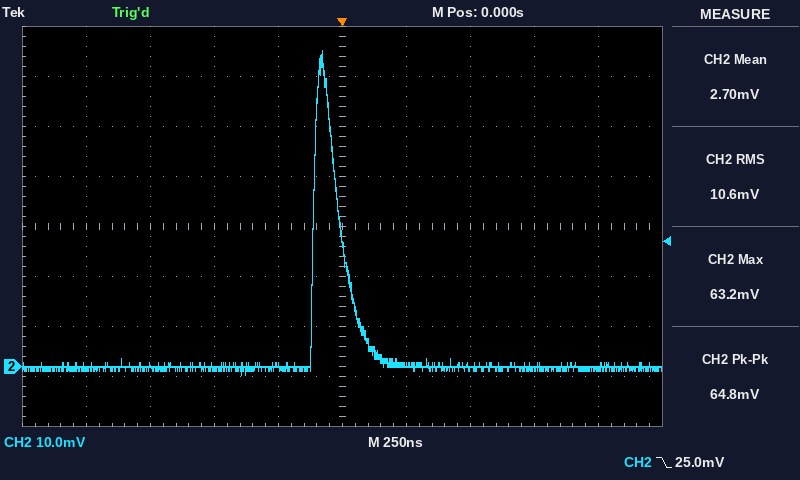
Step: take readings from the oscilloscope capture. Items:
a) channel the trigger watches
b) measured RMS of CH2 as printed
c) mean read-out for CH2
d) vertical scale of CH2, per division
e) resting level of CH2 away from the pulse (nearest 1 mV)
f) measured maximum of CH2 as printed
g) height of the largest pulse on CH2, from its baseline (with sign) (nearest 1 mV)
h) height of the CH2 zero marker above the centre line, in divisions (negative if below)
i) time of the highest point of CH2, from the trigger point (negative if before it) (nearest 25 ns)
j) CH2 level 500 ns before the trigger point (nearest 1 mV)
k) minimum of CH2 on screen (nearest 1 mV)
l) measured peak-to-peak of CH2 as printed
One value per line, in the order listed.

CH2
10.6 mV
2.70 mV
10 mV
0 mV
63.2 mV
+63 mV
-2.8 div
-75 ns
0 mV
-2 mV
64.8 mV
